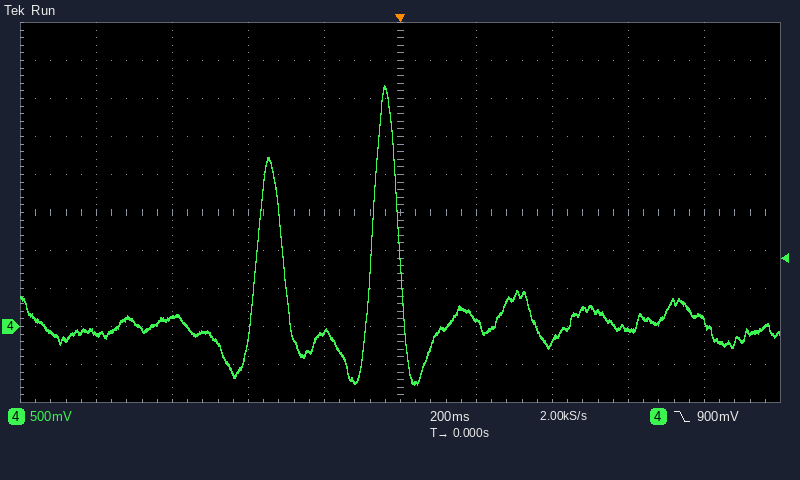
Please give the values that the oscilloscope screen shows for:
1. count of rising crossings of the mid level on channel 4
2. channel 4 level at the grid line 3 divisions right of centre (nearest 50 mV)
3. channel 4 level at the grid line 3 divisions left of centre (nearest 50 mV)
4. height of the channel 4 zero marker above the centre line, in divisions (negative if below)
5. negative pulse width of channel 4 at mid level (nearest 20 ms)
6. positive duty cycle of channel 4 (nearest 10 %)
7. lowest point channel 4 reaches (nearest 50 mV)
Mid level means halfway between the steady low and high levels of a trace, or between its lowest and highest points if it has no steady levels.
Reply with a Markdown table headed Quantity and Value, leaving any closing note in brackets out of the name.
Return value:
| Quantity | Value |
|---|---|
| count of rising crossings of the mid level on channel 4 | 2 |
| channel 4 level at the grid line 3 divisions right of centre | -50 mV |
| channel 4 level at the grid line 3 divisions left of centre | 100 mV |
| height of the channel 4 zero marker above the centre line, in divisions | -3.0 div |
| negative pulse width of channel 4 at mid level | 240 ms |
| positive duty cycle of channel 4 | 20 % |
| lowest point channel 4 reaches | -750 mV |
